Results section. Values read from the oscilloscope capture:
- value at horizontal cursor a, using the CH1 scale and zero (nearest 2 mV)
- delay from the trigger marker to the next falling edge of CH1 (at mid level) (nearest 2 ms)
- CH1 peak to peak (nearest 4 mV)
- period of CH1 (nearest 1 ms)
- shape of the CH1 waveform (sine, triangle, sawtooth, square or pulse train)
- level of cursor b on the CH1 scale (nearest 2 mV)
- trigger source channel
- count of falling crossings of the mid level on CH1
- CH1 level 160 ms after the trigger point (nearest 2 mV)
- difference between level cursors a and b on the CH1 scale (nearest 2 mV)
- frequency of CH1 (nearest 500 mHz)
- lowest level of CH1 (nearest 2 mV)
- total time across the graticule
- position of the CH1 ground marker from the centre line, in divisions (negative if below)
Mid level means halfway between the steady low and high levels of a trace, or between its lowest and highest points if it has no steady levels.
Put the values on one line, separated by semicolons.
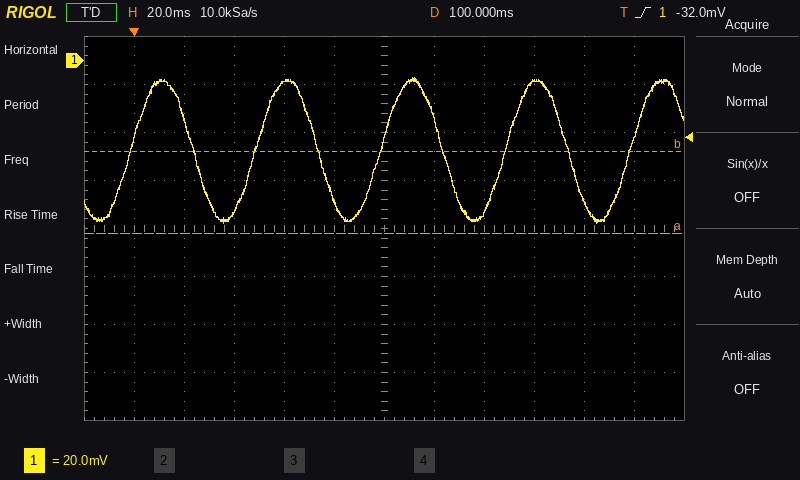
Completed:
-72 mV; 24 ms; 60 mV; 50 ms; sine; -38 mV; CH1; 4; -8 mV; 34 mV; 20.0 Hz; -68 mV; 240 ms; +3.5 div
